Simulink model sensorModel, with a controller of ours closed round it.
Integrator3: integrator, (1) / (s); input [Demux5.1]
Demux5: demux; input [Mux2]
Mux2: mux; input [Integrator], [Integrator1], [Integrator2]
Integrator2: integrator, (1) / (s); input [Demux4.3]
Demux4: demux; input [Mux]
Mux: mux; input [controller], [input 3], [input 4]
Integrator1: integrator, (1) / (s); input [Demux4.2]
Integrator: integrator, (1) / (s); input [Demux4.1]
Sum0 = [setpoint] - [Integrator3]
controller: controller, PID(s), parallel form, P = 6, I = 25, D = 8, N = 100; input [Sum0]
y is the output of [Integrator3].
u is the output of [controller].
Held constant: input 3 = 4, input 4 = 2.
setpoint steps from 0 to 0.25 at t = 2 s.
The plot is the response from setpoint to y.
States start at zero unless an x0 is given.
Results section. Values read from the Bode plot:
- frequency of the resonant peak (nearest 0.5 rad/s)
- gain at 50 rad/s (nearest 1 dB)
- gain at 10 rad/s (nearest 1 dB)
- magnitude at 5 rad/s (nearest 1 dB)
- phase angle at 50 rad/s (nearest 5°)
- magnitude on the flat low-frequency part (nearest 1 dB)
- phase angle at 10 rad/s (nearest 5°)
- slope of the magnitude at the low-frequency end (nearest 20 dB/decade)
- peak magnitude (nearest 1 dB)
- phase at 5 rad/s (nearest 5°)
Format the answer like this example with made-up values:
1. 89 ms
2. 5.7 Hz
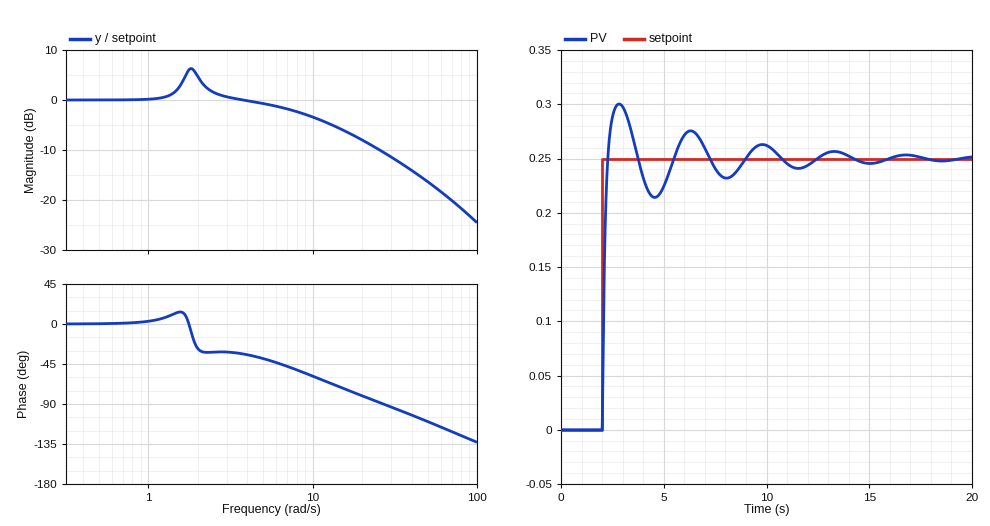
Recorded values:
1. 2.0 rad/s
2. -16 dB
3. -3 dB
4. -1 dB
5. -110°
6. 0 dB
7. -60°
8. 0 dB/decade
9. 6 dB
10. -40°
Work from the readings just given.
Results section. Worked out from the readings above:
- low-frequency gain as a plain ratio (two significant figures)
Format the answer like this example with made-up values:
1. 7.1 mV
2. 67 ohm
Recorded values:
1. 1.0
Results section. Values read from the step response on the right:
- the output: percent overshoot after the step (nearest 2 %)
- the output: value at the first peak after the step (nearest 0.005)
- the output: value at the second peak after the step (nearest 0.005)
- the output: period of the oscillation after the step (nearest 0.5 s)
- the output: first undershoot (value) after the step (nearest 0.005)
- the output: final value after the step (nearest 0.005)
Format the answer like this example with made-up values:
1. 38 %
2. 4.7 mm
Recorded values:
1. 20 %
2. 0.300
3. 0.275
4. 3.5 s
5. 0.215
6. 0.250
